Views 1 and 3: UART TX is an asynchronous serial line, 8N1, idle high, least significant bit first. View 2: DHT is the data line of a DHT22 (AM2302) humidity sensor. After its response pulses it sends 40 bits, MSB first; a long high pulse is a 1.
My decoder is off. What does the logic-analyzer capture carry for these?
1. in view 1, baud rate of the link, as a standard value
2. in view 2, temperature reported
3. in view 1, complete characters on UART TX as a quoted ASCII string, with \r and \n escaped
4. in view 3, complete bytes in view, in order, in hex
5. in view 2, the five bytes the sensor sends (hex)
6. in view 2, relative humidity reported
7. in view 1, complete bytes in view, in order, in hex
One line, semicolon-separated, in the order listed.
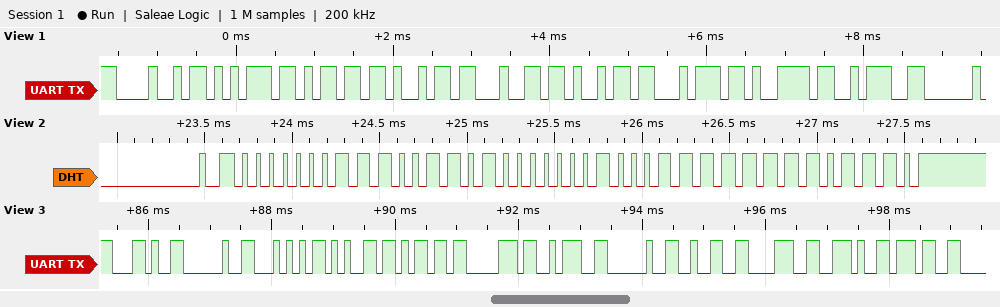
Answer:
9600 baud; 28.7 °C; "Humidity:"; 0x2C 0x20 0x54 0x65 0x6D 0x70 0x3A 0x20 0x32 0x38 0x2E 0x37; 01 CD 01 1F EE; 46.1 %; 0x48 0x75 0x6D 0x69 0x64 0x69 0x74 0x79 0x3A
